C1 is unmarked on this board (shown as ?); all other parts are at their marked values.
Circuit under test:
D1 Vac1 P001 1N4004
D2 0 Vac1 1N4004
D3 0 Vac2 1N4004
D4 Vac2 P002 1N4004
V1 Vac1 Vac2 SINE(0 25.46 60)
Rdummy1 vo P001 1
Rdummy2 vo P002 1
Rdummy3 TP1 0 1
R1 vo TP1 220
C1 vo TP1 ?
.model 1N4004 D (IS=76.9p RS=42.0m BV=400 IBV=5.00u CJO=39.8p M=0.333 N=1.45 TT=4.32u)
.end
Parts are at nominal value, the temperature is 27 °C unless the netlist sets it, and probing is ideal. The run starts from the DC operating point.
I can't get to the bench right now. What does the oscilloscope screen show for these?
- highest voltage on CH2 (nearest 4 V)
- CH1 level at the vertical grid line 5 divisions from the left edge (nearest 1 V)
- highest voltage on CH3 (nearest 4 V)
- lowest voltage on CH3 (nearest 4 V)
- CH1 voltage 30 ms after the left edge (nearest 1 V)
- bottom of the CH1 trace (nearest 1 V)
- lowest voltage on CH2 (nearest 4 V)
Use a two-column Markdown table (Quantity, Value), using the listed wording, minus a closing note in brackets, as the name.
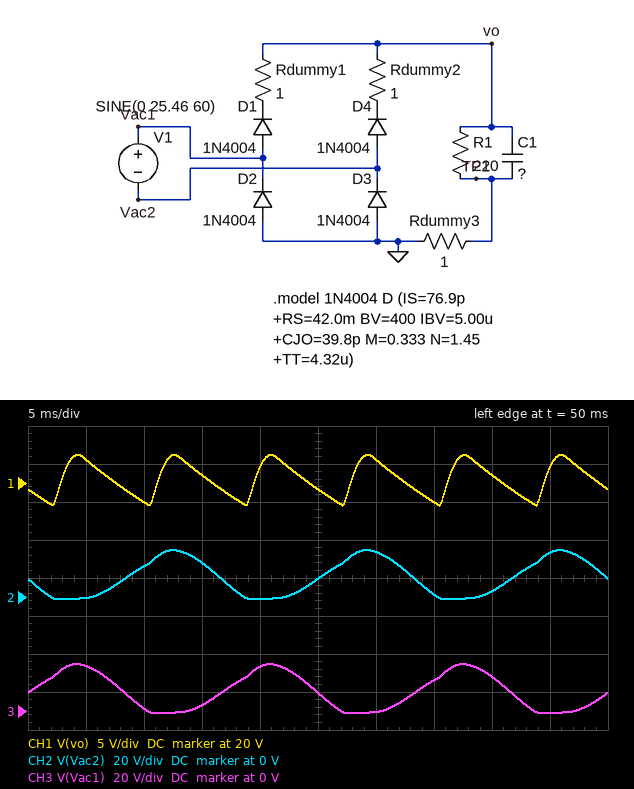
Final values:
| Quantity | Value |
|---|---|
| highest voltage on CH2 | 24 V |
| CH1 level at the vertical grid line 5 divisions from the left edge | 19 V |
| highest voltage on CH3 | 24 V |
| lowest voltage on CH3 | 0 V |
| CH1 voltage 30 ms after the left edge | 23 V |
| bottom of the CH1 trace | 17 V |
| lowest voltage on CH2 | 0 V |
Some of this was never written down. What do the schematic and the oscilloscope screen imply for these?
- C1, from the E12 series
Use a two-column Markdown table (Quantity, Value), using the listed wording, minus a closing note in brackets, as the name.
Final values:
| Quantity | Value |
|---|---|
| C1, from the E12 series | 82 µF |
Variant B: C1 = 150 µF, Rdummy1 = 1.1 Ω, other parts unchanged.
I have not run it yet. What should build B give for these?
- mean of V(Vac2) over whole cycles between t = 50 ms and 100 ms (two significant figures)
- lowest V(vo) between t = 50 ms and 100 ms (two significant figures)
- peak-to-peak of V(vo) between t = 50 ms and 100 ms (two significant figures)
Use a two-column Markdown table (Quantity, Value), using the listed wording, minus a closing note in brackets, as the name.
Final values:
| Quantity | Value |
|---|---|
| mean of V(Vac2) over whole cycles between t = 50 ms and 100 ms | 11 V |
| lowest V(vo) between t = 50 ms and 100 ms | 19 V |
| peak-to-peak of V(vo) between t = 50 ms and 100 ms | 4.2 V |
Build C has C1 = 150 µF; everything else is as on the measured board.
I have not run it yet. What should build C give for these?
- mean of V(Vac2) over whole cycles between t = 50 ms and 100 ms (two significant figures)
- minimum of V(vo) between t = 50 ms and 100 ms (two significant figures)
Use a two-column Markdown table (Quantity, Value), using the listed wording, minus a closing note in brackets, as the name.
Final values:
| Quantity | Value |
|---|---|
| mean of V(Vac2) over whole cycles between t = 50 ms and 100 ms | 11 V |
| minimum of V(vo) between t = 50 ms and 100 ms | 19 V |
